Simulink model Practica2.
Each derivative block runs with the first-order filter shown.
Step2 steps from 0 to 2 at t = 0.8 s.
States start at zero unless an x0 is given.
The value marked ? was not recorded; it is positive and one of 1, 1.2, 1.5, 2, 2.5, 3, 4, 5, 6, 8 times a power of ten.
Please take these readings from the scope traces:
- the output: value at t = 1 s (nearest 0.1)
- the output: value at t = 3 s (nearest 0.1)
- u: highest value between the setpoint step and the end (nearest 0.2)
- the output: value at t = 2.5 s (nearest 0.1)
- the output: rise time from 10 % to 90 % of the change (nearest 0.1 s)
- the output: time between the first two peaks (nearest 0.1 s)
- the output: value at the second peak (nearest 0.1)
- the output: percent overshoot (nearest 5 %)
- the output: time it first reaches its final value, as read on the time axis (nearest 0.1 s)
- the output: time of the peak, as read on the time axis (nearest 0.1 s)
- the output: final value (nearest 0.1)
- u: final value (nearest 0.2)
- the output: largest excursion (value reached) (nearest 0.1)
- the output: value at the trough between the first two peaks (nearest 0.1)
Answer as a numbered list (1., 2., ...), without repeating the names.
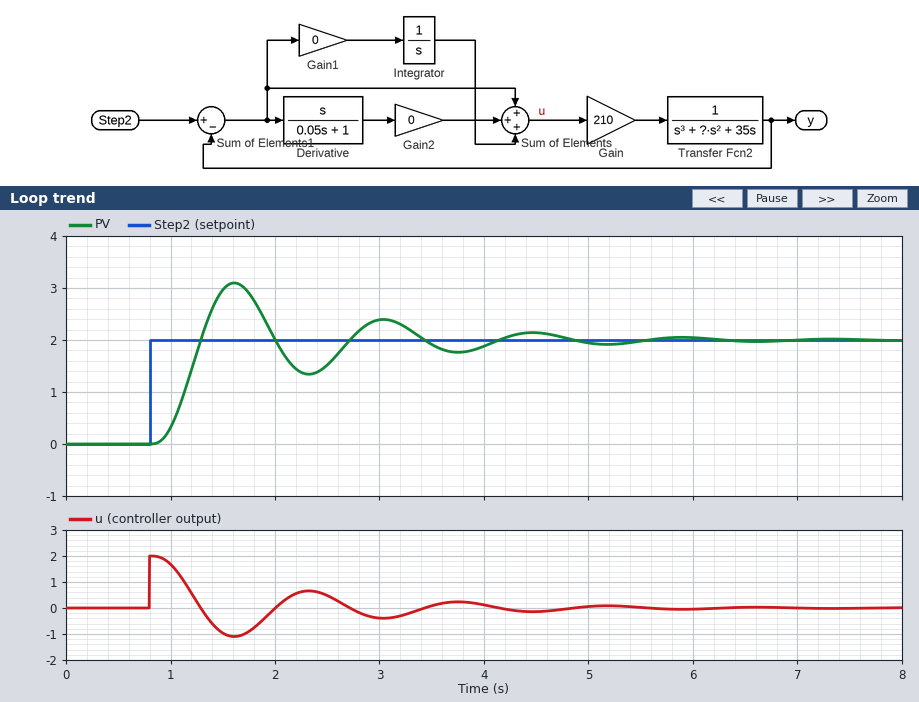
1. 0.3
2. 2.4
3. 2.0
4. 1.5
5. 0.3 s
6. 1.4 s
7. 2.4
8. 55 %
9. 1.3 s
10. 1.6 s
11. 2.0
12. 0.0
13. 3.1
14. 1.3
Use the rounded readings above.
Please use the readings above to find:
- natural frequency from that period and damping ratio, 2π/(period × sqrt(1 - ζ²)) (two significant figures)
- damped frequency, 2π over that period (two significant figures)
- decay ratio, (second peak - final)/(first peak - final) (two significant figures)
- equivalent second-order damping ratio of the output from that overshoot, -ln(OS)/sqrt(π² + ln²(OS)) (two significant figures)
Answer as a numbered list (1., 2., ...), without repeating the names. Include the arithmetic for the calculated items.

1. 2π / (1.4 × sqrt(1 - 0.19²)) = 4.6 rad/s
2. 2π / 1.4 = 4.5 rad/s
3. (2.4 - 2) / (3.1 - 2) = 0.36
4. ln(0.55) = -0.598; 0.598 / sqrt(9.870 + 0.357) = 0.19
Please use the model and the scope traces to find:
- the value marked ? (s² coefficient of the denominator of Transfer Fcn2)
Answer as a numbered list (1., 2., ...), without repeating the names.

1. 12
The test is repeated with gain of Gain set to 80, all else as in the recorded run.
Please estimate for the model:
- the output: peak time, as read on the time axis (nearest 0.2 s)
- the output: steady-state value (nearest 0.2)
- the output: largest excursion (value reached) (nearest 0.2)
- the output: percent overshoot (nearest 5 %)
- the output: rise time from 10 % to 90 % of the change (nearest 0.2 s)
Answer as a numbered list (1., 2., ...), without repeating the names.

1. 2.2 s
2. 2.0
3. 2.4
4. 15 %
5. 0.6 s
